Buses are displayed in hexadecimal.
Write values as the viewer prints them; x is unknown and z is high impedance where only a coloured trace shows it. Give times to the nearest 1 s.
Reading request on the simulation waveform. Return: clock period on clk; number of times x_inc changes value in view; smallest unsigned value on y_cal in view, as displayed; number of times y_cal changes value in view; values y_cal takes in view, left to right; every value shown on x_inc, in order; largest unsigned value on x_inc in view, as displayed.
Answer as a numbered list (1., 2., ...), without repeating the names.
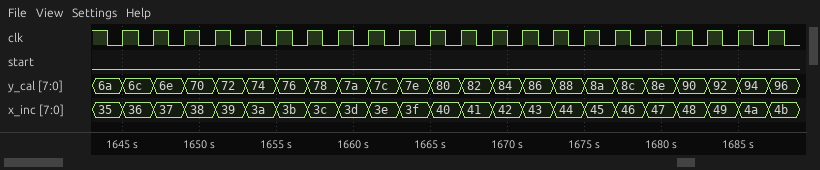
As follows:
1. 2 s
2. 22
3. 6a
4. 22
5. 6a, 6c, 6e, 70, 72, 74, 76, 78, 7a, 7c, 7e, 80, 82, 84, 86, 88, 8a, 8c, 8e, 90, 92, 94, 96
6. 35, 36, 37, 38, 39, 3a, 3b, 3c, 3d, 3e, 3f, 40, 41, 42, 43, 44, 45, 46, 47, 48, 49, 4a, 4b
7. 4b
